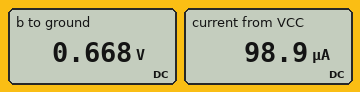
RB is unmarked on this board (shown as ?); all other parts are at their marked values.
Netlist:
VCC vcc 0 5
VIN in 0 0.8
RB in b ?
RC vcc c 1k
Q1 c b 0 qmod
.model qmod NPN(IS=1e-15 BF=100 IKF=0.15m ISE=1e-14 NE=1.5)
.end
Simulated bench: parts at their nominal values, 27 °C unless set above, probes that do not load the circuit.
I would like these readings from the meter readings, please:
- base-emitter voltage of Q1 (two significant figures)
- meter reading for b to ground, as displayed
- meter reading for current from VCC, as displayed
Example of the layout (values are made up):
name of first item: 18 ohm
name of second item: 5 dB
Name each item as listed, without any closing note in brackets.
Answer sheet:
base-emitter voltage of Q1: 670 mV
meter reading for b to ground, as displayed: 0.668 V
meter reading for current from VCC, as displayed: 98.9 µA
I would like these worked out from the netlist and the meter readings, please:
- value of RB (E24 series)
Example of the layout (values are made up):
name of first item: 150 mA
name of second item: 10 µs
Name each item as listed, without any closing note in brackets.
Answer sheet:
value of RB: 68 kΩ
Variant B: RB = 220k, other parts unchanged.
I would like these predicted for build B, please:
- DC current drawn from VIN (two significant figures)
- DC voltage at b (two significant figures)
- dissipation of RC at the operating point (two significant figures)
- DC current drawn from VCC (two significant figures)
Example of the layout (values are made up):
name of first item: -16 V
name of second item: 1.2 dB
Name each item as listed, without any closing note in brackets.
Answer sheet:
DC current drawn from VIN: 720 nA
DC voltage at b: 640 mV
dissipation of RC at the operating point: 2.0 µW
DC current drawn from VCC: 44 µA
